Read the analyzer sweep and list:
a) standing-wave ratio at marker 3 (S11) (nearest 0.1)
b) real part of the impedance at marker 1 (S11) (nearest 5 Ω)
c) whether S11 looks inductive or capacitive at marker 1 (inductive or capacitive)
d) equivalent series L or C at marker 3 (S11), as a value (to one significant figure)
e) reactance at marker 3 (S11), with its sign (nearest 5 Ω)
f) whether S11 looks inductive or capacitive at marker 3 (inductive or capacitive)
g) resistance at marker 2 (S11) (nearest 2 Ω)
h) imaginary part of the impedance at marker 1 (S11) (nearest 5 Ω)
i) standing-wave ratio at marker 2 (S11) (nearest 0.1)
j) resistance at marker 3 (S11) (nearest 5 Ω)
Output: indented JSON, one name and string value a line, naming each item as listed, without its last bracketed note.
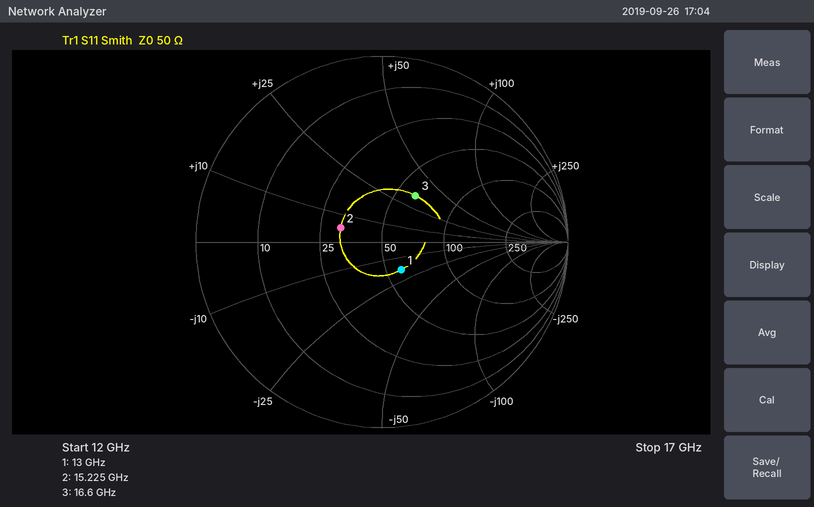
{
  "standing-wave ratio at marker 3 (S11)": "1.9",
  "real part of the impedance at marker 1 (S11)": "60 Ω",
  "whether S11 looks inductive or capacitive at marker 1": "capacitive",
  "equivalent series L or C at marker 3 (S11), as a value": "300 pH",
  "reactance at marker 3 (S11), with its sign": "+35 Ω",
  "whether S11 looks inductive or capacitive at marker 3": "inductive",
  "resistance at marker 2 (S11)": "32 Ω",
  "imaginary part of the impedance at marker 1 (S11)": "-20 Ω",
  "standing-wave ratio at marker 2 (S11)": "1.6",
  "resistance at marker 3 (S11)": "60 Ω"
}
